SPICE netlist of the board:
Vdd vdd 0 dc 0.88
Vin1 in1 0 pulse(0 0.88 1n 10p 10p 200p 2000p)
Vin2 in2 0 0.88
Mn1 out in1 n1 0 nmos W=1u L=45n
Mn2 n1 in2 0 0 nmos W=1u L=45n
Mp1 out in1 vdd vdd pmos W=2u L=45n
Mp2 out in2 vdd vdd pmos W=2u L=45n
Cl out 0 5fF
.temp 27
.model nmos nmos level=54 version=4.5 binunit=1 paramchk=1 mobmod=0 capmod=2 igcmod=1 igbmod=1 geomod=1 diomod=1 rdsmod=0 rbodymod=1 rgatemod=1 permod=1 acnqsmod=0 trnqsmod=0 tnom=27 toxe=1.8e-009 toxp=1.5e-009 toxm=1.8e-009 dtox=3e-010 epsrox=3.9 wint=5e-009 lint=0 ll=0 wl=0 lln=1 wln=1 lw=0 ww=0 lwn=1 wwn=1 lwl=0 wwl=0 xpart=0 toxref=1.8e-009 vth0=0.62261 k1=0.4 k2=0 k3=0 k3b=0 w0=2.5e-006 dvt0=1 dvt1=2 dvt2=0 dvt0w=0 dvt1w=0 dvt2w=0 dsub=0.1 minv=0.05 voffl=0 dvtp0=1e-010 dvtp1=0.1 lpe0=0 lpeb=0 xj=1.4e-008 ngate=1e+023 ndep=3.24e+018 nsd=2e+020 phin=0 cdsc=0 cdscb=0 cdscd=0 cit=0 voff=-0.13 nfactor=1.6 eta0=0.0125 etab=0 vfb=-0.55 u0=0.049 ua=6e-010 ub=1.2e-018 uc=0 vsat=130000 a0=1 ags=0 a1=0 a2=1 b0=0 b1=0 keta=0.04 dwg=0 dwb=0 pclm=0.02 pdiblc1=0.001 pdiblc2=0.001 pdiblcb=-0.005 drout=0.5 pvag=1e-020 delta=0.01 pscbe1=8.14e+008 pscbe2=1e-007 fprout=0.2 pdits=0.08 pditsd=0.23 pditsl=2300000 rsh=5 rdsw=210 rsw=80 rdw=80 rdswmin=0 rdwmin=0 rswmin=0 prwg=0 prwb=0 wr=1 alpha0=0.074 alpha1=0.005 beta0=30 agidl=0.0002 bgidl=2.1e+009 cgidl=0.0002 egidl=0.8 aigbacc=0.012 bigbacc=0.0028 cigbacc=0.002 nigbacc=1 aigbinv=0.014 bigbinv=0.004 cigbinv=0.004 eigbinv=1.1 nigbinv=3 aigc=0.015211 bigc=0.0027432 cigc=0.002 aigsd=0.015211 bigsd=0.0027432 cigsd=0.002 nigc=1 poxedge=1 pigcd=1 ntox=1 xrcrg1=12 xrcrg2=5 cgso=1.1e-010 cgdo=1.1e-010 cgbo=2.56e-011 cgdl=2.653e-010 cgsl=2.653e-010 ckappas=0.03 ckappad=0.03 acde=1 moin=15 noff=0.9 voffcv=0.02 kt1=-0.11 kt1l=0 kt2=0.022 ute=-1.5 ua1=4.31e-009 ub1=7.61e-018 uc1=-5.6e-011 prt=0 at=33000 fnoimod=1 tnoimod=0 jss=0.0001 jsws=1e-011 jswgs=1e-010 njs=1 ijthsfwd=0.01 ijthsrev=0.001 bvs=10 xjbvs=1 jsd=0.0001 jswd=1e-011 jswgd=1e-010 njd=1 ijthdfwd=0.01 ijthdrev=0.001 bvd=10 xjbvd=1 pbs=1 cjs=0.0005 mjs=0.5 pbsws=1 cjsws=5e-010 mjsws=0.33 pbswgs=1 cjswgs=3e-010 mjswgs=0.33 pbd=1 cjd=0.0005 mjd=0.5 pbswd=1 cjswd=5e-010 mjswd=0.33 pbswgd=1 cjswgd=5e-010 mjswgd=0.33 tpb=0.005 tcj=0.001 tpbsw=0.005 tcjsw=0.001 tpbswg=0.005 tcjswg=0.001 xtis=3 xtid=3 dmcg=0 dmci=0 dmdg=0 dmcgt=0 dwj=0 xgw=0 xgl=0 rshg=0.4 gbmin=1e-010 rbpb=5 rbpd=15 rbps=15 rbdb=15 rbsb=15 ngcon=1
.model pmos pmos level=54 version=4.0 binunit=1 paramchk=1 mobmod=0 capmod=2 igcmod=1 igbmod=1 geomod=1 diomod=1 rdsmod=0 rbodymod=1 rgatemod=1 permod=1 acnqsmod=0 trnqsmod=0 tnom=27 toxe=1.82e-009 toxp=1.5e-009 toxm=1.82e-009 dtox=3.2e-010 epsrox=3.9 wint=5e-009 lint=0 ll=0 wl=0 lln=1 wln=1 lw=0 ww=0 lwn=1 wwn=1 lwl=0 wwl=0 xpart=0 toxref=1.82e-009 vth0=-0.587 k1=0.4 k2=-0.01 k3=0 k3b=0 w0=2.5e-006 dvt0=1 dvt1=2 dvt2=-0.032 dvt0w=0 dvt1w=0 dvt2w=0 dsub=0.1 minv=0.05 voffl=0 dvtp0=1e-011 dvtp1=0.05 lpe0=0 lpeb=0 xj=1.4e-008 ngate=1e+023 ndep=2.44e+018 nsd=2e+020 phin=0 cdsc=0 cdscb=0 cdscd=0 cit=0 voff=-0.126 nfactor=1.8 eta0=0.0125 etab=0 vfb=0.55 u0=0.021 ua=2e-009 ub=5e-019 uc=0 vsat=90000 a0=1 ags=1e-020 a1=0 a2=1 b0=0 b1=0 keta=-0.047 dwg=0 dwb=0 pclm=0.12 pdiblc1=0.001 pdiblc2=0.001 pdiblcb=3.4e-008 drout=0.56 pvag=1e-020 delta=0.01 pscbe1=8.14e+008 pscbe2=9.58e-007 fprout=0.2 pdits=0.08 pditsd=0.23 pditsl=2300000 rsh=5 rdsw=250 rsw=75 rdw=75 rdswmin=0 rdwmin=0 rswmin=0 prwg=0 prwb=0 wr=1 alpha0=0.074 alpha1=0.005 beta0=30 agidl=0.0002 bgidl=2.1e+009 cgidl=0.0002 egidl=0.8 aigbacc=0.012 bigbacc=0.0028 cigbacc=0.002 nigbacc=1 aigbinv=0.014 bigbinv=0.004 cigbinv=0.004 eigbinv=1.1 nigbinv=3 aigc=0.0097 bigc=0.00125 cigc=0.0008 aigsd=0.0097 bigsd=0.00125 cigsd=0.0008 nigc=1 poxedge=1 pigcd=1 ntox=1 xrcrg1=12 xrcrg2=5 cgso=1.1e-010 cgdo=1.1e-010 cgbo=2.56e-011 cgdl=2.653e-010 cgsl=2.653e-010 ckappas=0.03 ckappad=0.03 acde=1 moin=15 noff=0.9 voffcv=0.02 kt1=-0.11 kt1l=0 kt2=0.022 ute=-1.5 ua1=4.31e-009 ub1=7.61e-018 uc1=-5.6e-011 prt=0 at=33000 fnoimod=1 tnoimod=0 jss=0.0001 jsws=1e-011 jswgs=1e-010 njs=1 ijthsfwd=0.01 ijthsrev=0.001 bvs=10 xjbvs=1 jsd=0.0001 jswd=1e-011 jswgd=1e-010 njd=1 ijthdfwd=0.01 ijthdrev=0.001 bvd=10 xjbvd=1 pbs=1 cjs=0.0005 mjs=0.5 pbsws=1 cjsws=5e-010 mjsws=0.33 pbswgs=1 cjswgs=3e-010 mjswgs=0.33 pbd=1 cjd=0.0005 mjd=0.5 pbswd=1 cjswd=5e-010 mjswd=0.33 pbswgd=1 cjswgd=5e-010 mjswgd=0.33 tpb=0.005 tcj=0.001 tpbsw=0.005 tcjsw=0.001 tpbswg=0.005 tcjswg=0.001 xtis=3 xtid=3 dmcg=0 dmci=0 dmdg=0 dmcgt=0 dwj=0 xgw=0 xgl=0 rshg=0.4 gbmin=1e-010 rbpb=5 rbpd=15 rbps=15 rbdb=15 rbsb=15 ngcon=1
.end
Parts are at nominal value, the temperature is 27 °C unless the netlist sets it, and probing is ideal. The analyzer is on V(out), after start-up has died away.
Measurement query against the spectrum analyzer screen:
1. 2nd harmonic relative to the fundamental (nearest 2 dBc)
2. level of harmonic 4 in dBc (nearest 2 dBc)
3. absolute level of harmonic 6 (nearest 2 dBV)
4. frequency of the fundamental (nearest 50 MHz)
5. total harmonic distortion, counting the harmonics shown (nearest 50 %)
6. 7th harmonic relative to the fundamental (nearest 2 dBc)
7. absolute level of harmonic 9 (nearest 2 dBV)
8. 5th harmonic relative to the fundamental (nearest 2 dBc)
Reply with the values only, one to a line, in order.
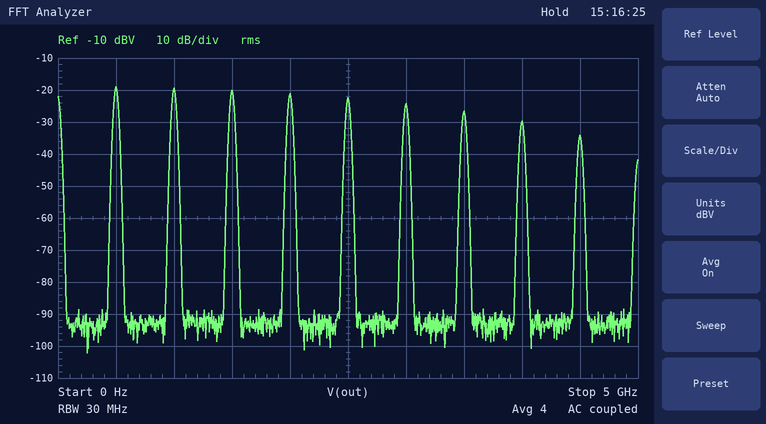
0 dBc
-2 dBc
-24 dBV
500 MHz
200 %
-8 dBc
-34 dBV
-4 dBc
